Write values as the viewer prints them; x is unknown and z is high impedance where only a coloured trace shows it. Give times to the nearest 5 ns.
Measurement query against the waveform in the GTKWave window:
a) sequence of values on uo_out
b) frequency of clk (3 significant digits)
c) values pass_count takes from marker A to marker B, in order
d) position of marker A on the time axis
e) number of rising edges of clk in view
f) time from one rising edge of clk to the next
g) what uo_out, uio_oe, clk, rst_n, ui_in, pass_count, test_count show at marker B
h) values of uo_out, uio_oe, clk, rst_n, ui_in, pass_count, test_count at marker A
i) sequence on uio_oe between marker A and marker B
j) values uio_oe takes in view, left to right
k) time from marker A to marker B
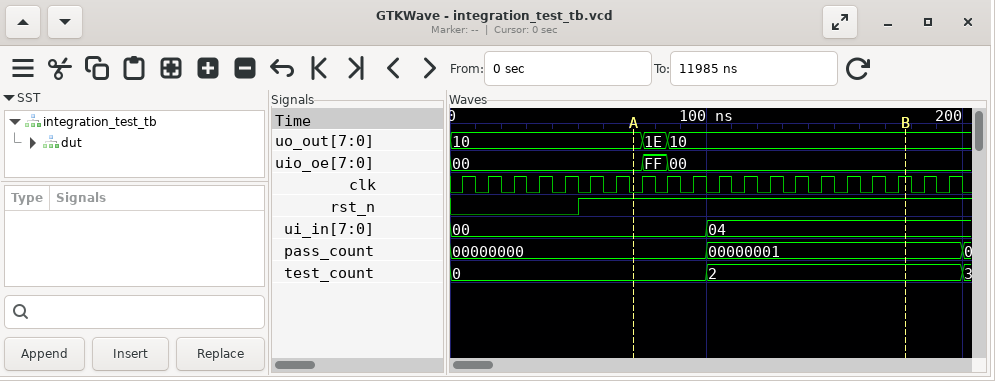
10, 1E, 10
100 MHz
00000000, 00000001
70 ns
20
10 ns
uo_out=10, uio_oe=00, clk=1, rst_n=1, ui_in=04, pass_count=00000001, test_count=2
uo_out=10, uio_oe=00, clk=0, rst_n=1, ui_in=00, pass_count=00000000, test_count=0
00, FF, 00
00, FF, 00
105 ns
